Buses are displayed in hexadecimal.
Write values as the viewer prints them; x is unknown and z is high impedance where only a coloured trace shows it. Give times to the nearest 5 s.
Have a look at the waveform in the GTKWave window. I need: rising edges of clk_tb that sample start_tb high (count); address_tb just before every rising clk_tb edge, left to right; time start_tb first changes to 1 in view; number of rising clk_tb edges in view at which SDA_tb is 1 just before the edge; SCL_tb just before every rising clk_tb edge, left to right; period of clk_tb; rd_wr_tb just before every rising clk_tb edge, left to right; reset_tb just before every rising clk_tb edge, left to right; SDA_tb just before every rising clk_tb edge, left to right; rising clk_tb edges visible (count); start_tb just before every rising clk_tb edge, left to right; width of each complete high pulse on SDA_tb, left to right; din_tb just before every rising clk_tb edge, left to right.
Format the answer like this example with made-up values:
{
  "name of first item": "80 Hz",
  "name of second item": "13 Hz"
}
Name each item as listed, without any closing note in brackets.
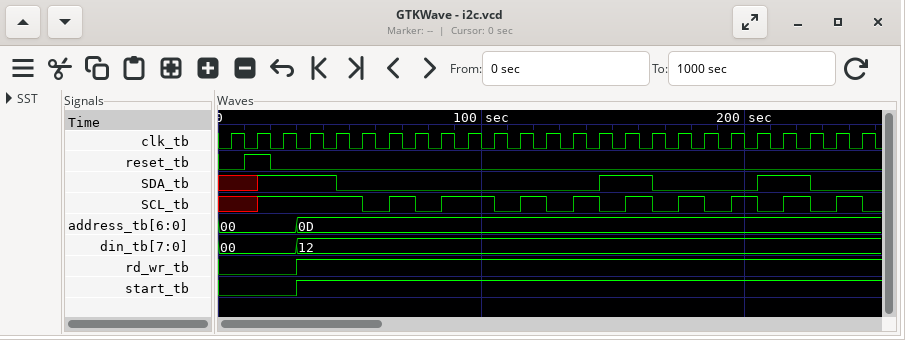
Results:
{
  "rising edges of clk_tb that sample start_tb high": "22",
  "address_tb just before every rising clk_tb edge, left to right": "00, 00, 00, 0D, 0D, 0D, 0D, 0D, 0D, 0D, 0D, 0D, 0D, 0D, 0D, 0D, 0D, 0D, 0D, 0D, 0D, 0D, 0D, 0D, 0D",
  "time start_tb first changes to 1 in view": "30 s",
  "number of rising clk_tb edges in view at which SDA_tb is 1 just before the edge": "7",
  "SCL_tb just before every rising clk_tb edge, left to right": "x x 1 1 1 1 0 1 0 1 1 0 1 0 1 0 1 0 1 0 1 0 1 0 1",
  "period of clk_tb": "10 s",
  "rd_wr_tb just before every rising clk_tb edge, left to right": "0 0 0 1 1 1 1 1 1 1 1 1 1 1 1 1 1 1 1 1 1 1 1 1 1",
  "reset_tb just before every rising clk_tb edge, left to right": "0 1 0 0 0 0 0 0 0 0 0 0 0 0 0 0 0 0 0 0 0 0 0 0 0",
  "SDA_tb just before every rising clk_tb edge, left to right": "x x 1 1 1 0 0 0 0 0 0 0 0 0 0 1 1 0 0 0 0 1 1 0 0",
  "rising clk_tb edges visible": "25",
  "start_tb just before every rising clk_tb edge, left to right": "0 0 0 1 1 1 1 1 1 1 1 1 1 1 1 1 1 1 1 1 1 1 1 1 1",
  "width of each complete high pulse on SDA_tb, left to right": "20 s, 20 s",
  "din_tb just before every rising clk_tb edge, left to right": "00, 00, 00, 12, 12, 12, 12, 12, 12, 12, 12, 12, 12, 12, 12, 12, 12, 12, 12, 12, 12, 12, 12, 12, 12"
}
